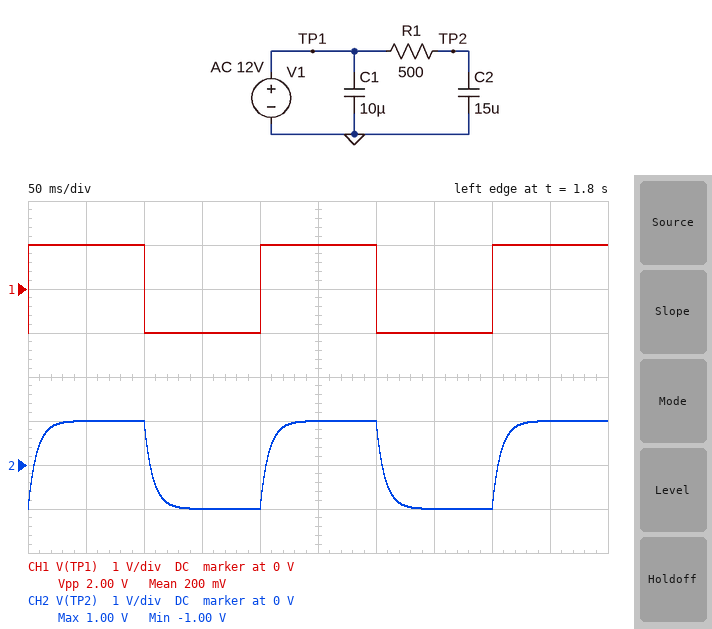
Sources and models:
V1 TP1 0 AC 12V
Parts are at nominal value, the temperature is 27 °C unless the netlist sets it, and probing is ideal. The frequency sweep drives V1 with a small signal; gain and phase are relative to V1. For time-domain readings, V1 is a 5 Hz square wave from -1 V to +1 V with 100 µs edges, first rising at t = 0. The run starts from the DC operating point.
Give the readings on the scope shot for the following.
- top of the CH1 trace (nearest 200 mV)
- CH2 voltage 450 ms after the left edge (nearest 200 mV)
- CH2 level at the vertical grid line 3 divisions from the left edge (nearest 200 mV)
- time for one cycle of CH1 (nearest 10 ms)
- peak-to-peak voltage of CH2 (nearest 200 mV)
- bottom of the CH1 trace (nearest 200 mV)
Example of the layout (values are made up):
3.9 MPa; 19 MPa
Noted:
1.0 V; 1.0 V; -1.0 V; 200 ms; 2.0 V; -1.0 V
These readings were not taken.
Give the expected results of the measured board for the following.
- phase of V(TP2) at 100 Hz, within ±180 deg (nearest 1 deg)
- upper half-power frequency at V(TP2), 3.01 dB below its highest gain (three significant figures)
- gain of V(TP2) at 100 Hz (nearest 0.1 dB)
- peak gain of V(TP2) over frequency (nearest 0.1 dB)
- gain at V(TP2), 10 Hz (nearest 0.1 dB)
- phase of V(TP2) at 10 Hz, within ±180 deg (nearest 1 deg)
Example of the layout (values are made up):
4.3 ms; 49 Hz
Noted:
-78 deg; 21.2 Hz; -13.7 dB; 0 dB; -0.9 dB; -25 deg
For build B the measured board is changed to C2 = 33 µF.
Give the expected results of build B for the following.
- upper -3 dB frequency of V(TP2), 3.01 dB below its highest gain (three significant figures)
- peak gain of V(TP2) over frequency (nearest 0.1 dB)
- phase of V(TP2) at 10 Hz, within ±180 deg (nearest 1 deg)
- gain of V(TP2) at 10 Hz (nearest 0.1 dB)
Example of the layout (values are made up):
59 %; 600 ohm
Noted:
9.65 Hz; 0 dB; -46 deg; -3.2 dB
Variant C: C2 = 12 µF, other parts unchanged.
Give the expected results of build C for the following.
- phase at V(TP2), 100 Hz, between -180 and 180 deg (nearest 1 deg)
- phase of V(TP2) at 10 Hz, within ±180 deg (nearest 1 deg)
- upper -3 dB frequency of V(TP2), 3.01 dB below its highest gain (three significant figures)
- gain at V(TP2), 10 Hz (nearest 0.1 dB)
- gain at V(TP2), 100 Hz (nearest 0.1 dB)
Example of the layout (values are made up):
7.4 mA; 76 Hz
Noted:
-75 deg; -21 deg; 26.5 Hz; -0.6 dB; -11.8 dB
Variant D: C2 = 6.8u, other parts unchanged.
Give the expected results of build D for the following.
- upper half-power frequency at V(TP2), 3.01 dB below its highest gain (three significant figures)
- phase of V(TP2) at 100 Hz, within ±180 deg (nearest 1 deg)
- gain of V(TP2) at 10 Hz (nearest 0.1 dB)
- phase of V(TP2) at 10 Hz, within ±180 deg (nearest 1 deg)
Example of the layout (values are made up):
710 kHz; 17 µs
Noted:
46.8 Hz; -65 deg; -0.2 dB; -12 deg
